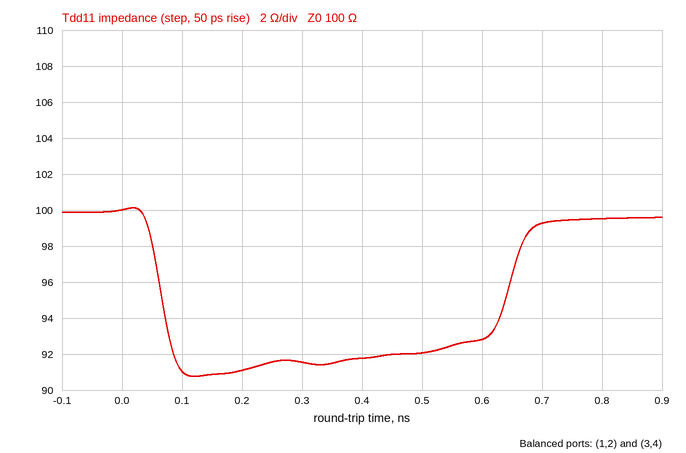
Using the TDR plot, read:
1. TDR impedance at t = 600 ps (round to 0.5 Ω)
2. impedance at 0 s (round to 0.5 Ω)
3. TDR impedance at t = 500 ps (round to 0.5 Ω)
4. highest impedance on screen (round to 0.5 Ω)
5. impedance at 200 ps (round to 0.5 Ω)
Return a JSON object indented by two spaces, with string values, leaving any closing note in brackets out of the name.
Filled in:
{
  "TDR impedance at t = 600 ps": "93.0 Ω",
  "impedance at 0 s": "100.0 Ω",
  "TDR impedance at t = 500 ps": "92.0 Ω",
  "highest impedance on screen": "100.0 Ω",
  "impedance at 200 ps": "91.0 Ω"
}
